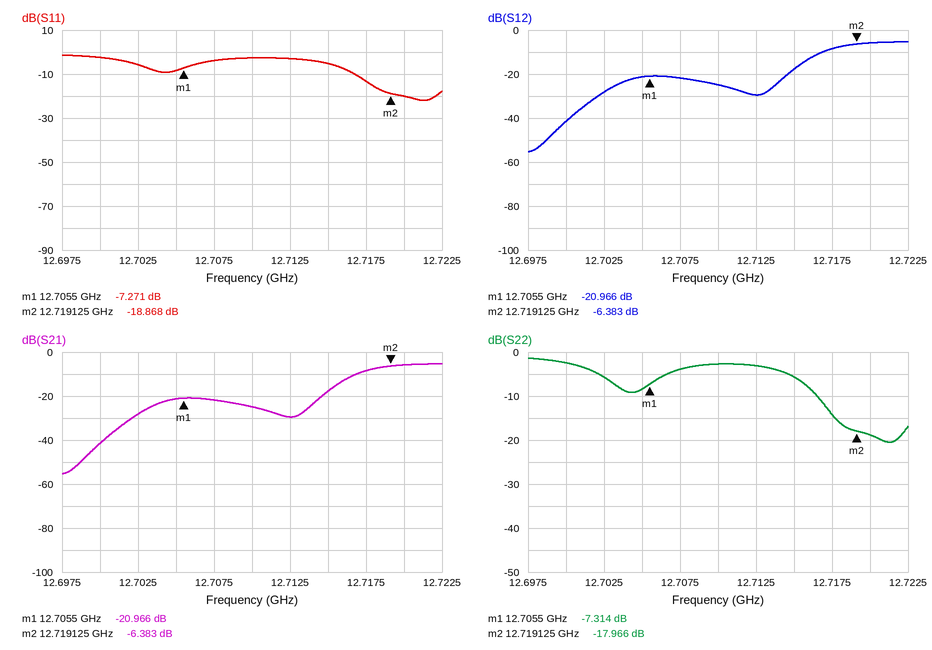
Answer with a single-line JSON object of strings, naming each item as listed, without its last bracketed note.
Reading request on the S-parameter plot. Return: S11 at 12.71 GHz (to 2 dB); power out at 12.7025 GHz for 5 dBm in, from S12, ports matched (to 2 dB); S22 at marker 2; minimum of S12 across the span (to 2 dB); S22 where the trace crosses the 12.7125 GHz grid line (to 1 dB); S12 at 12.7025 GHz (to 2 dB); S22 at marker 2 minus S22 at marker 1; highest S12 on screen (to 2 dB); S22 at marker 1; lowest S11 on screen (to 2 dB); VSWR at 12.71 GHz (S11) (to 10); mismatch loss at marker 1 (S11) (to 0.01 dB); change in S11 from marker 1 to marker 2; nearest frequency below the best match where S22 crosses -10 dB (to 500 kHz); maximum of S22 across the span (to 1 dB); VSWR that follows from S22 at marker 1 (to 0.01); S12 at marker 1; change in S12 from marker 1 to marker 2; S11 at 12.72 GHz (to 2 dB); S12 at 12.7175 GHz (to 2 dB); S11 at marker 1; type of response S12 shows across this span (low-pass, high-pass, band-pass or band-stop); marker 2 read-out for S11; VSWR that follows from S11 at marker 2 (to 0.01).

{"S11 at 12.71 GHz": "-2 dB", "power out at 12.7025 GHz for 5 dBm in, from S12, ports matched": "-24 dBm", "S22 at marker 2": "-17.966 dB", "minimum of S12 across the span": "-56 dB", "S22 where the trace crosses the 12.7125 GHz grid line": "-3 dB", "S12 at 12.7025 GHz": "-28 dB", "S22 at marker 2 minus S22 at marker 1": "-10.652 dB", "highest S12 on screen": "-6 dB", "S22 at marker 1": "-7.314 dB", "lowest S11 on screen": "-22 dB", "VSWR at 12.71 GHz (S11)": "10", "mismatch loss at marker 1 (S11)": "0.90 dB", "change in S11 from marker 1 to marker 2": "-11.597 dB", "nearest frequency below the best match where S22 crosses -10 dB": "12.7165 GHz", "maximum of S22 across the span": "-1 dB", "VSWR that follows from S22 at marker 1": "2.51", "S12 at marker 1": "-20.966 dB", "change in S12 from marker 1 to marker 2": "14.583 dB", "S11 at 12.72 GHz": "-20 dB", "S12 at 12.7175 GHz": "-8 dB", "S11 at marker 1": "-7.271 dB", "type of response S12 shows across this span": "high-pass", "marker 2 read-out for S11": "-18.868 dB", "VSWR that follows from S11 at marker 2": "1.26"}
